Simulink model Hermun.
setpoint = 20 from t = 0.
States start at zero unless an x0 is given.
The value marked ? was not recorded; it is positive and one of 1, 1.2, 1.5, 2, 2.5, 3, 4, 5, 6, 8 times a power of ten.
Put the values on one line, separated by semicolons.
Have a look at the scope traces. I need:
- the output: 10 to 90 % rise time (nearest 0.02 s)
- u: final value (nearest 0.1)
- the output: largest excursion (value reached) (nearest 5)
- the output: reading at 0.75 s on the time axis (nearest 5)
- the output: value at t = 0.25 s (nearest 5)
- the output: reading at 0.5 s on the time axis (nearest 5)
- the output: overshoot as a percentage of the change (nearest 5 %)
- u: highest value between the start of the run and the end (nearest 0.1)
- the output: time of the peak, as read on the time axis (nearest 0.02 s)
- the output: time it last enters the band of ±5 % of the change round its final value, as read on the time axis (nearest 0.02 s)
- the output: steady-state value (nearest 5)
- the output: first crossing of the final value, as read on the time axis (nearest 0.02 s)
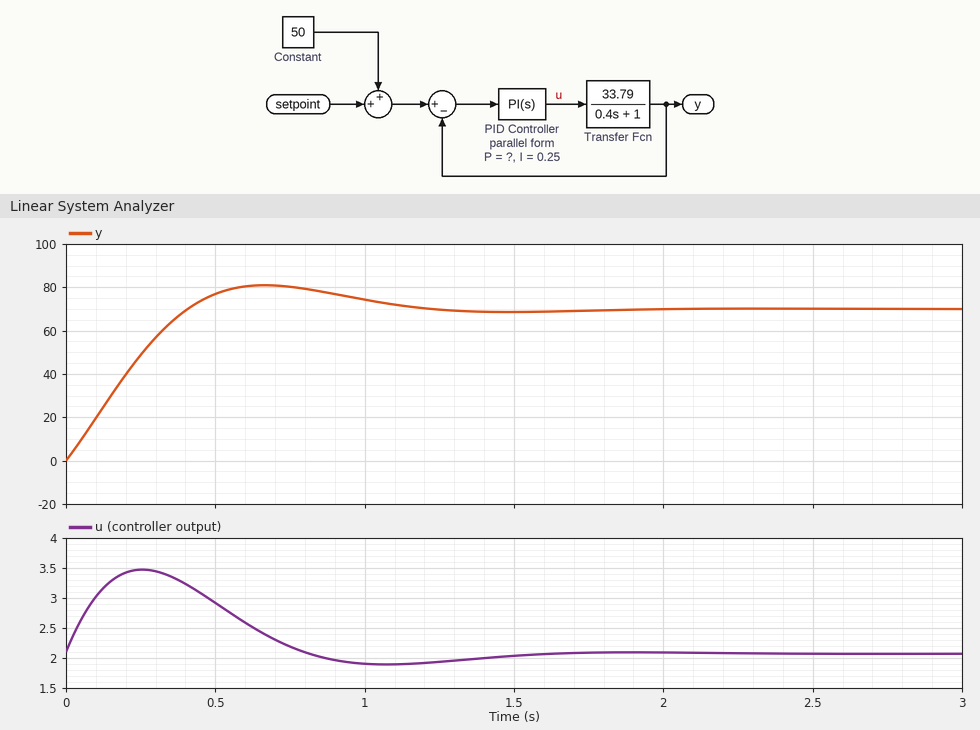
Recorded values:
0.30 s; 2.1; 80; 80; 50; 75; 15 %; 3.5; 0.66 s; 1.04 s; 70; 0.40 s
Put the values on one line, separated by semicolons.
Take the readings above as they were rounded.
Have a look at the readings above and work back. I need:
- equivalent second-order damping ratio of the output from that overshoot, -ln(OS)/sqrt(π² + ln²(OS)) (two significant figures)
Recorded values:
0.52
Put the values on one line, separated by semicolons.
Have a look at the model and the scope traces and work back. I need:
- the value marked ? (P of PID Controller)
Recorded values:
0.03
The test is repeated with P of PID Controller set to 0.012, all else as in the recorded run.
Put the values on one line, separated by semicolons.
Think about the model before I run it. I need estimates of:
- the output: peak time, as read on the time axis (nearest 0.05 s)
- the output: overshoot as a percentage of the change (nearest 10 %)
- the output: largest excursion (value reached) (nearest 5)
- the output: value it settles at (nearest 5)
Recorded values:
0.70 s; 30 %; 90; 70
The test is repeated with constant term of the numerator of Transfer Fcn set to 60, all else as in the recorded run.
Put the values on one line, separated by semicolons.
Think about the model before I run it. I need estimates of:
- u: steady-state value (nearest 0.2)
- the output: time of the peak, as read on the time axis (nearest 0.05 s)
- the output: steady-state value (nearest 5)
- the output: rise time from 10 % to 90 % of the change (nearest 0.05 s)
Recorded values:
1.2; 0.45 s; 70; 0.20 s
